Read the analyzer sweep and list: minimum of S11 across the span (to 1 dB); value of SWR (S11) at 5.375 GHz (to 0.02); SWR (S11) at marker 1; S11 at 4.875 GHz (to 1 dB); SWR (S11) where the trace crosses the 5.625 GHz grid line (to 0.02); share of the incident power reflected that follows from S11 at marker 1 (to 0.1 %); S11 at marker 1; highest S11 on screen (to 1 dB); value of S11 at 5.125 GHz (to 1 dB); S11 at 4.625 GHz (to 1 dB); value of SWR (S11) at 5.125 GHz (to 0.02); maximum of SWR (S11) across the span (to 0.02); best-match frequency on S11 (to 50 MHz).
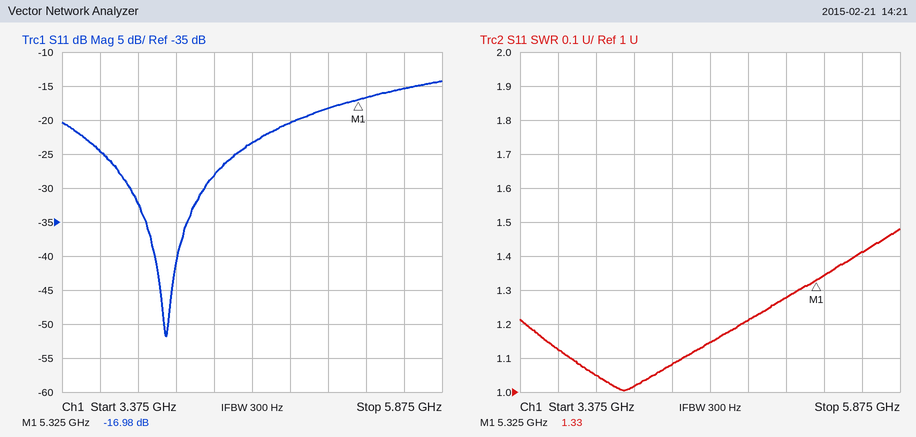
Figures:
-52 dB
1.34
1.33
-20 dB
1.42
2.0 %
-16.98 dB
-14 dB
-18 dB
-23 dB
1.28
1.48
4.05 GHz
